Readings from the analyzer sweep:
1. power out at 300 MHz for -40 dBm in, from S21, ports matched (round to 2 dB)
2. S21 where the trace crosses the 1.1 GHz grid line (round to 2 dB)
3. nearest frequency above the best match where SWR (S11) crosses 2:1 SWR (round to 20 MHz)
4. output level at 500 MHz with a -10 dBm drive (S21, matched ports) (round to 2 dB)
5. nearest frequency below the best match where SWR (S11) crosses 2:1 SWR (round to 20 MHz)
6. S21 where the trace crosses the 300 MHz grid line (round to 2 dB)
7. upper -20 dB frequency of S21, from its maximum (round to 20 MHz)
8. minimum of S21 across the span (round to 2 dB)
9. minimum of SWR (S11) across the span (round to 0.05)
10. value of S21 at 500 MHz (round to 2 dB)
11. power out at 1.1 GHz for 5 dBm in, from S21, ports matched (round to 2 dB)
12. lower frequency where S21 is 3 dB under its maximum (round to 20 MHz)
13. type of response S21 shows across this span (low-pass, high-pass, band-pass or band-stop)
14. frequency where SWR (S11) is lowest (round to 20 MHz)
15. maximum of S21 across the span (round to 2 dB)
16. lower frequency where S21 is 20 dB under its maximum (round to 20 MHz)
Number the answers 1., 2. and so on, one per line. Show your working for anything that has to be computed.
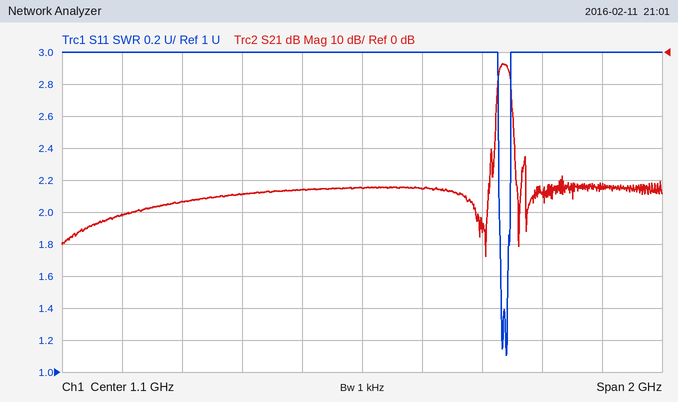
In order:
1. -40 dBm + (-50 dB) = -90 dBm
2. -42 dB
3. 1.60 GHz
4. -10 dBm + (-46 dB) = -56 dBm
5. 1.56 GHz
6. -50 dB
7. 1.60 GHz
8. -64 dB
9. 1.10
10. -46 dB
11. 5 dBm + (-42 dB) = -38 dBm
12. 1.56 GHz
13. band-pass
14. 1.58 GHz
15. -4 dB
16. 1.54 GHz
